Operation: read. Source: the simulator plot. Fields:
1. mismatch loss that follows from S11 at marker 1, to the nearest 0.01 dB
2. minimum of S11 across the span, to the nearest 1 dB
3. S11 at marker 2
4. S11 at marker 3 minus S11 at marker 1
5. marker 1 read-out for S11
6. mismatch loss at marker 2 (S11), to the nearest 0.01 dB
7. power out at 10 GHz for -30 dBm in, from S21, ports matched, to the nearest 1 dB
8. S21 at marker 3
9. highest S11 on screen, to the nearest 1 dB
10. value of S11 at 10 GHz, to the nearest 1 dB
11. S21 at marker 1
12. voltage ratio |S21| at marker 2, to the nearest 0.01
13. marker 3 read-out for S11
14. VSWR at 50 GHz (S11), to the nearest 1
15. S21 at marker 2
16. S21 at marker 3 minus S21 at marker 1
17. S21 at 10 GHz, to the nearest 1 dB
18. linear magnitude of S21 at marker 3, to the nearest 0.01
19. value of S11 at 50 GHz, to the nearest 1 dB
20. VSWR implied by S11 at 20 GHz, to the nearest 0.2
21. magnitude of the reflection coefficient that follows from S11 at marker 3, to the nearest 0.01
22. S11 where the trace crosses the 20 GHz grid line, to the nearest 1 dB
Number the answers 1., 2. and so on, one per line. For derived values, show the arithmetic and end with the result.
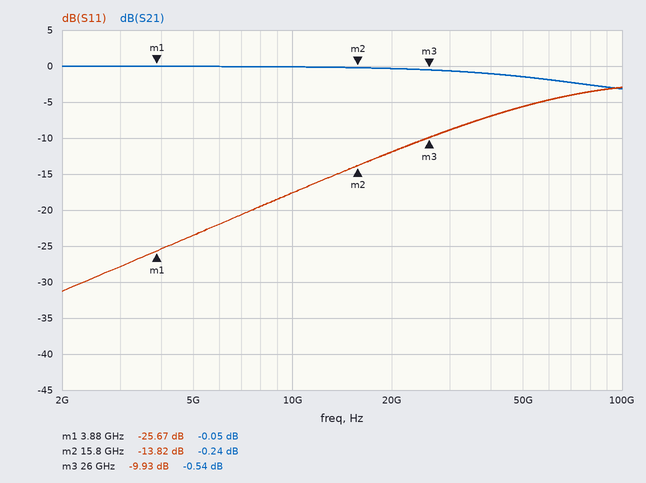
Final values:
1. −10 log10(1 − 10^(-25.67/10)) ≈ 0.01 dB
2. -31 dB
3. -13.82 dB
4. -9.93 − (-25.67) = 15.74 dB
5. -25.67 dB
6. −10 log10(1 − 10^(-13.82/10)) ≈ 0.18 dB
7. -30 dBm + (0 dB) = -30 dBm
8. -0.54 dB
9. -3 dB
10. -18 dB
11. -0.05 dB
12. 10^(-0.24/20) ≈ 0.97
13. -9.93 dB
14. |Γ| = 10^(-6/20) = 0.5012; VSWR = (1 + 0.5012)/(1 − 0.5012) ≈ 3
15. -0.24 dB
16. -0.54 − (-0.05) = -0.49 dB
17. 0 dB
18. 10^(-0.54/20) ≈ 0.94
19. -6 dB
20. |Γ| = 10^(-12/20) = 0.2512; VSWR = (1 + 0.2512)/(1 − 0.2512) ≈ 1.67, so 1.6 to the nearest 0.2
21. 10^(-9.93/20) ≈ 0.32
22. -12 dB
